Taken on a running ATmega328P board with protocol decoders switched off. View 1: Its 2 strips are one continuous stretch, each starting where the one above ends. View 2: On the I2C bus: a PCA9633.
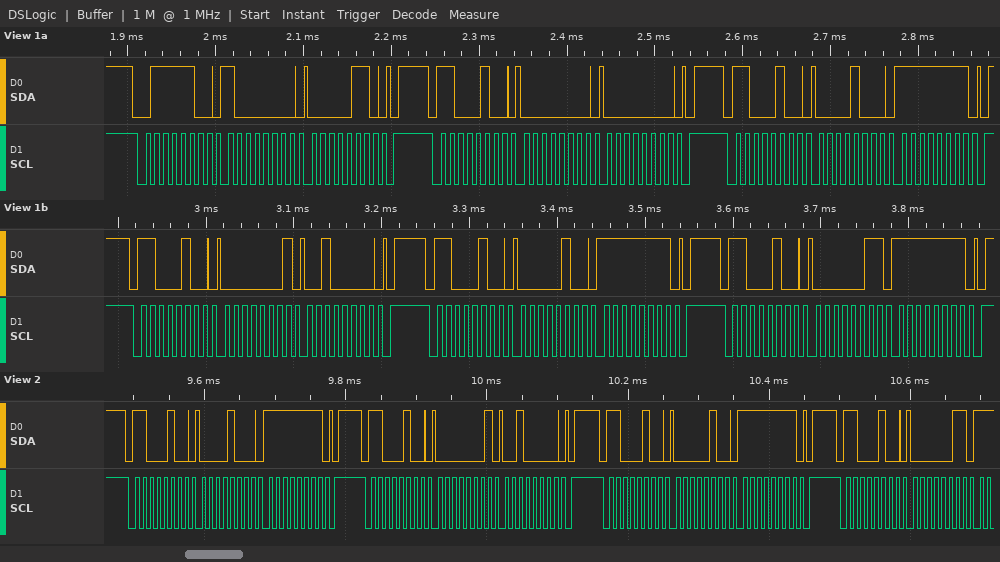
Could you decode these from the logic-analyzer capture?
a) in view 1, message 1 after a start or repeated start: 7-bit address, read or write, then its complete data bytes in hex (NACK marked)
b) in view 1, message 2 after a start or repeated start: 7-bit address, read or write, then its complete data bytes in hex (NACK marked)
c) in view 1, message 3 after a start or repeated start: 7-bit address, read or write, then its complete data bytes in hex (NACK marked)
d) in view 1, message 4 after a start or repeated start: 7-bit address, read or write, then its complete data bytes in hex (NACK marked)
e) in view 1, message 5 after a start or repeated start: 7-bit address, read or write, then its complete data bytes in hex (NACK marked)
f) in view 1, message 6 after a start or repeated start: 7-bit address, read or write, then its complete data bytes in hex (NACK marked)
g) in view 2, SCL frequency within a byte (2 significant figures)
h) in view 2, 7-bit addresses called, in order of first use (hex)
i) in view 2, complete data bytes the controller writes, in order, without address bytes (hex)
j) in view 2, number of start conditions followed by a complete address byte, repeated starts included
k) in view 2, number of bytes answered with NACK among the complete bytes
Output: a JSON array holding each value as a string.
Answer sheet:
["0x3E write: 80 06", "0x62 write: 00 00", "0x62 write: 08 FF", "0x62 write: 01 20", "0x62 write: 04 FF", "0x62 write: 03 FF", "100 kHz", "0x62", "08 FF 01 20 04 FF 03", "4", "0"]
